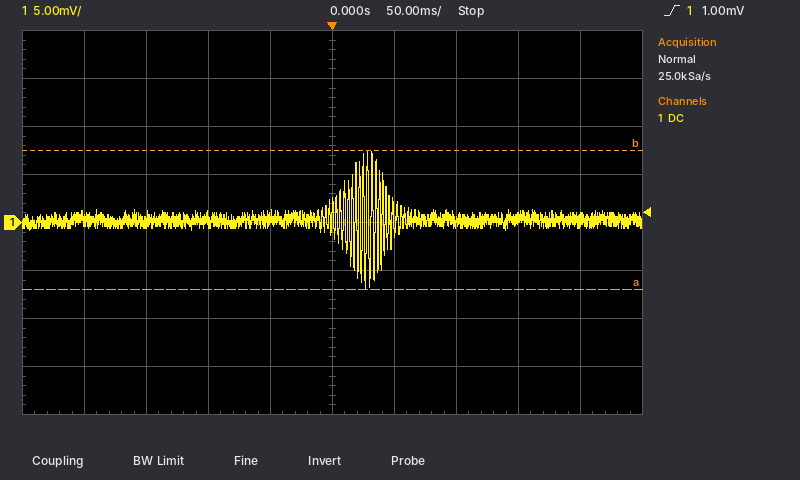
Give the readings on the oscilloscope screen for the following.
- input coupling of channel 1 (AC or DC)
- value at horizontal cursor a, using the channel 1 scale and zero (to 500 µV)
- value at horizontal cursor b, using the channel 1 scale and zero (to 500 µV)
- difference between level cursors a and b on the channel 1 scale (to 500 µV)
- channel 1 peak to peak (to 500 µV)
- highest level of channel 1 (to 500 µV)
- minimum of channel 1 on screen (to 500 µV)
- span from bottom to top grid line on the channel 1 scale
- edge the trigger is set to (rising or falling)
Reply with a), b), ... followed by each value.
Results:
a) DC
b) -7.0 mV
c) 7.5 mV
d) 14.5 mV
e) 14.5 mV
f) 7.5 mV
g) -7.0 mV
h) 40 mV
i) rising
